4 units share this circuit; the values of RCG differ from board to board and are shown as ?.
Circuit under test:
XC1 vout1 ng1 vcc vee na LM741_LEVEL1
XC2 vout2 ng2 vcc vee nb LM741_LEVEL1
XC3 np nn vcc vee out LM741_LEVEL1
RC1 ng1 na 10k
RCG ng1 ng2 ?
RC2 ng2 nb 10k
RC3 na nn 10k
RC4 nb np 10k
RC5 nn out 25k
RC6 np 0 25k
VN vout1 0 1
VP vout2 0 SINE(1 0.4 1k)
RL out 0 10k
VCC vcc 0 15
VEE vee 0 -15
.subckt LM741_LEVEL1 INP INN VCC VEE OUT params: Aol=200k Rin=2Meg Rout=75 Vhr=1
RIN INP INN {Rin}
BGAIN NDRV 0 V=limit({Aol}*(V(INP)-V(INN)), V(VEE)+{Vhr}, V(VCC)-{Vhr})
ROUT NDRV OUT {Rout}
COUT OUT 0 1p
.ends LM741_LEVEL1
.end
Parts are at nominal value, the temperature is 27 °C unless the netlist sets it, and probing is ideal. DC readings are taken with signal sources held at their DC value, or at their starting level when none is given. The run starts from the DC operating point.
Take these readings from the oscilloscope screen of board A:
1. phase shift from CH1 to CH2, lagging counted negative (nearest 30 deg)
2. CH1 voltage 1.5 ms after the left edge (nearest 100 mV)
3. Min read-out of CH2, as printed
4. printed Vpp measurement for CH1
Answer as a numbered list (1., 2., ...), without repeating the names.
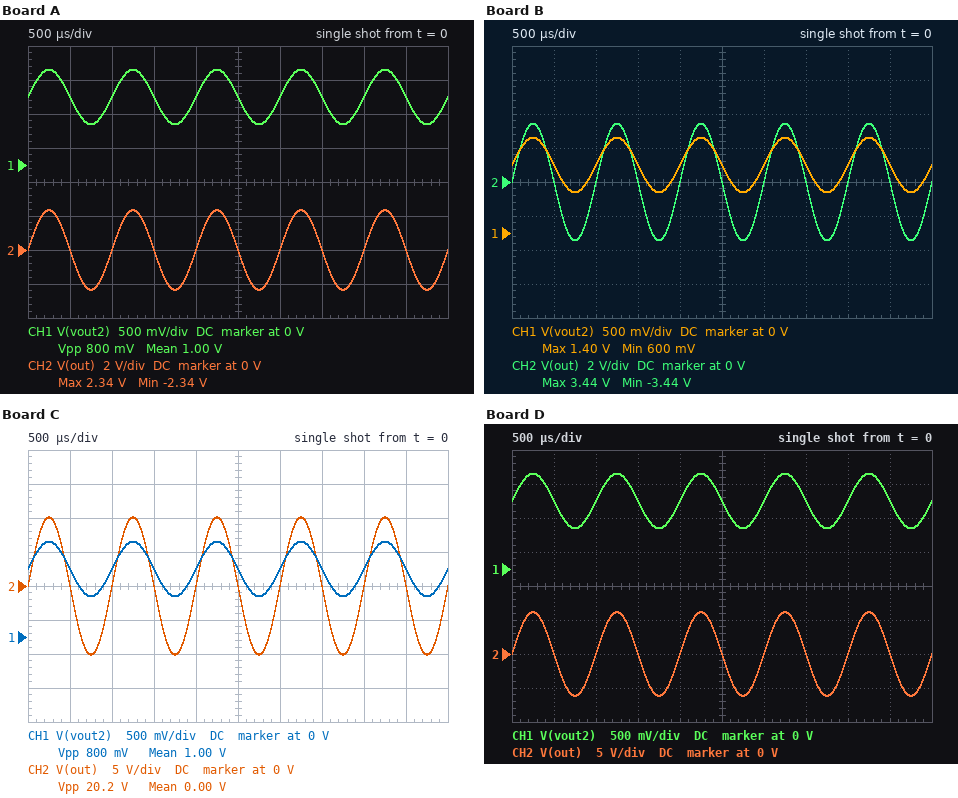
1. 0 deg
2. 1.0 V
3. -2.34 V
4. 800 mV
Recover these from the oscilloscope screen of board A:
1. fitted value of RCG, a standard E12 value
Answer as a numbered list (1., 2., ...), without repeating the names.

1. 15 kΩ
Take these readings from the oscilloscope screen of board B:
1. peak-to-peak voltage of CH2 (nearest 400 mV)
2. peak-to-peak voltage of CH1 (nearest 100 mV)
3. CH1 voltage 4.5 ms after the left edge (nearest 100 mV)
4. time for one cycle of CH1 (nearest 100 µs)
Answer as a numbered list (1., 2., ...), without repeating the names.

1. 6.8 V
2. 800 mV
3. 1.0 V
4. 1.0 ms
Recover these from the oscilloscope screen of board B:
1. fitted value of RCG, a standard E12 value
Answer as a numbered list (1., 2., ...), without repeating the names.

1. 8.2 kΩ
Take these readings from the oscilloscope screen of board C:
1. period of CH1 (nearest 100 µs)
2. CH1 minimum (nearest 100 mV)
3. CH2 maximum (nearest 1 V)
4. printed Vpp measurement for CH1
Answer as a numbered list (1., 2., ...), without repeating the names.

1. 1.0 ms
2. 600 mV
3. 10 V
4. 800 mV
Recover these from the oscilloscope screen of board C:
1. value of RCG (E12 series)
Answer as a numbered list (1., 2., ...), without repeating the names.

1. 2.2 kΩ
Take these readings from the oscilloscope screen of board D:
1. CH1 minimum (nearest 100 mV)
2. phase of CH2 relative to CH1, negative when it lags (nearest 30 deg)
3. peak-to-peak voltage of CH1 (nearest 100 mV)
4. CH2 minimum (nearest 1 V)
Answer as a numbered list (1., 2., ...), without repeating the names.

1. 600 mV
2. 0 deg
3. 800 mV
4. -6 V
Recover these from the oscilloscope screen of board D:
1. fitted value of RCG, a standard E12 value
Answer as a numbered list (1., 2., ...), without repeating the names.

1. 3.9 kΩ
